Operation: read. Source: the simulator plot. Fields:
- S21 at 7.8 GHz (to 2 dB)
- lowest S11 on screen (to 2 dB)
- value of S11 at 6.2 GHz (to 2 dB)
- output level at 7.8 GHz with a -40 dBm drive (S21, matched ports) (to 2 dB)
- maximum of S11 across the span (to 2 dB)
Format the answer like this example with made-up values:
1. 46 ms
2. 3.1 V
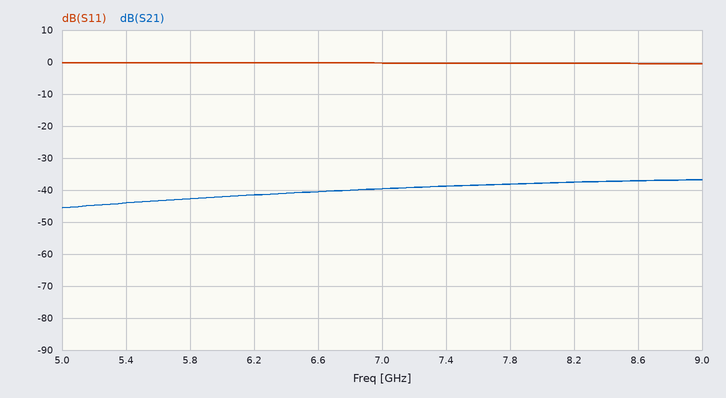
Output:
1. -38 dB
2. 0 dB
3. 0 dB
4. -78 dBm
5. 0 dB
